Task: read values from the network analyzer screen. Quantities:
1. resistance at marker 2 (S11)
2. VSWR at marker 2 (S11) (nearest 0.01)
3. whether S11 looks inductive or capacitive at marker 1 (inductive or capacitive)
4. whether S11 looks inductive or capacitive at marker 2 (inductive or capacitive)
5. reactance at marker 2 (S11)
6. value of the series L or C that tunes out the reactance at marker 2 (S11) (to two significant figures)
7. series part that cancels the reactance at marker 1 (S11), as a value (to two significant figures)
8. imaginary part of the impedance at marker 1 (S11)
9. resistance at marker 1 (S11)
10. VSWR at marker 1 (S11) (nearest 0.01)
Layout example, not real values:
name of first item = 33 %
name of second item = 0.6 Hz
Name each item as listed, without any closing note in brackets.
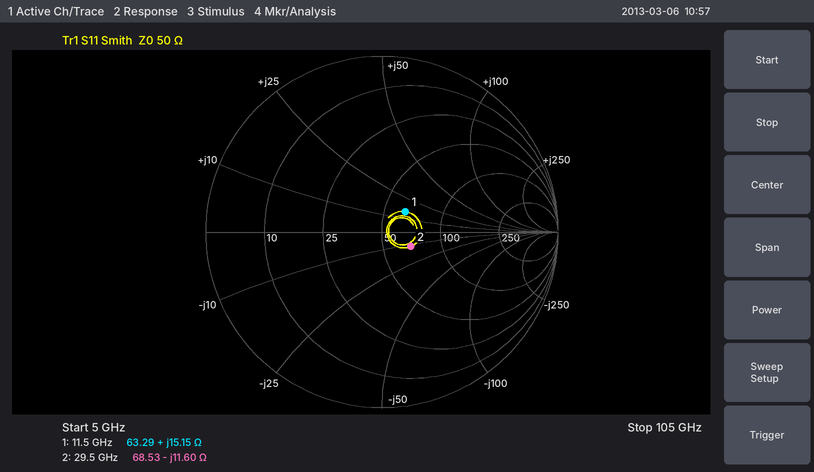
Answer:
resistance at marker 2 = 68.53 Ω
VSWR at marker 2 (S11) = 1.45
whether S11 looks inductive or capacitive at marker 1 = inductive
whether S11 looks inductive or capacitive at marker 2 = capacitive
reactance at marker 2 = -11.60 Ω
value of the series L or C that tunes out the reactance at marker 2 (S11) = 63 pH
series part that cancels the reactance at marker 1 (S11), as a value = 910 fF
imaginary part of the impedance at marker 1 = +15.15 Ω
resistance at marker 1 = 63.29 Ω
VSWR at marker 1 (S11) = 1.43
